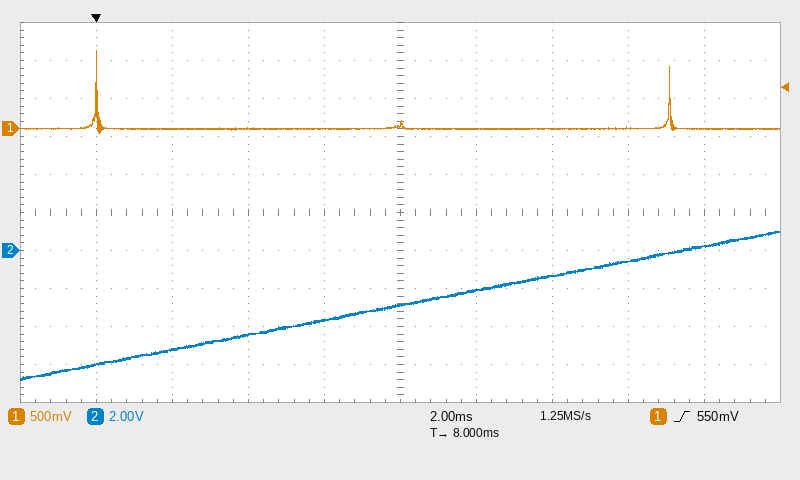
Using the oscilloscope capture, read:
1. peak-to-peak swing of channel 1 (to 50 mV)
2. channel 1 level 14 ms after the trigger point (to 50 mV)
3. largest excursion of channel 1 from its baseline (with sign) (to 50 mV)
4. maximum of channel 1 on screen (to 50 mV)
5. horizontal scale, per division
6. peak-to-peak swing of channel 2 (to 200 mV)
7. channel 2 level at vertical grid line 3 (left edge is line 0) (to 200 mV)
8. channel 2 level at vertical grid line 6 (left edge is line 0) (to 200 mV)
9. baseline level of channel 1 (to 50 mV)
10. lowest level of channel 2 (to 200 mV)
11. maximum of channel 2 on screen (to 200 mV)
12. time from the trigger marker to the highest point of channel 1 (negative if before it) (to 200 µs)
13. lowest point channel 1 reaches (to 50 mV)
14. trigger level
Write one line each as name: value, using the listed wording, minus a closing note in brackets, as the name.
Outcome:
peak-to-peak swing of channel 1: 1.10 V
channel 1 level 14 ms after the trigger point: 0 mV
largest excursion of channel 1 from its baseline (with sign): +1.05 V
maximum of channel 1 on screen: 1.05 V
horizontal scale, per division: 2 ms
peak-to-peak swing of channel 2: 7.8 V
channel 2 level at vertical grid line 3 (left edge is line 0): -4.4 V
channel 2 level at vertical grid line 6 (left edge is line 0): -2.2 V
baseline level of channel 1: 0 mV
lowest level of channel 2: -6.8 V
maximum of channel 2 on screen: 1.0 V
time from the trigger marker to the highest point of channel 1 (negative if before it): 0.0 ms
lowest point channel 1 reaches: -50 mV
trigger level: 550 mV
